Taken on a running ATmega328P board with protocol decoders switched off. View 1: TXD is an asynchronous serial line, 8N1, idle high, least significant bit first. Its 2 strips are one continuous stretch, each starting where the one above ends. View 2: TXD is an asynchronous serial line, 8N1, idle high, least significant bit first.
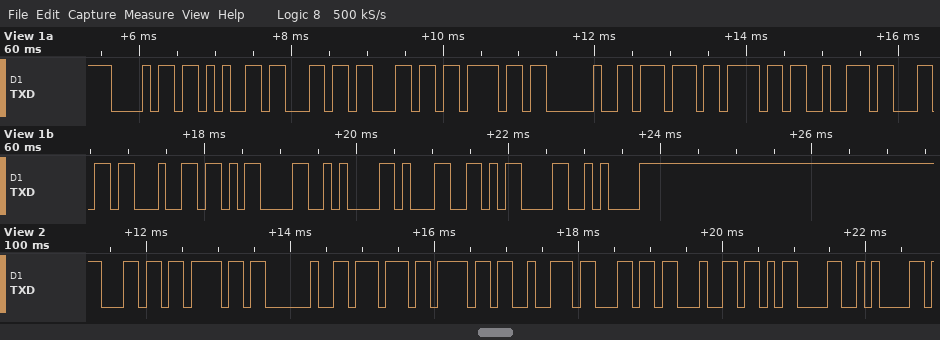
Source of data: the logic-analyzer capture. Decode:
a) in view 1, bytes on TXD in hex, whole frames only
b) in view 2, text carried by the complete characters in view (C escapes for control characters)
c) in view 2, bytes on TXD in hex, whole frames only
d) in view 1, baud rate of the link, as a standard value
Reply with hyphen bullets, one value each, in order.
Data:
- 0x68 0x65 0x6C 0x6C 0x6F 0x20 0x77 0x6F 0x72 0x6C 0x64 0x0D 0x0A 0x31 0x0D 0x0A
- "lo world\r\n"
- 6C 6F 20 77 6F 72 6C 64 0D 0A
- 9600 baud
